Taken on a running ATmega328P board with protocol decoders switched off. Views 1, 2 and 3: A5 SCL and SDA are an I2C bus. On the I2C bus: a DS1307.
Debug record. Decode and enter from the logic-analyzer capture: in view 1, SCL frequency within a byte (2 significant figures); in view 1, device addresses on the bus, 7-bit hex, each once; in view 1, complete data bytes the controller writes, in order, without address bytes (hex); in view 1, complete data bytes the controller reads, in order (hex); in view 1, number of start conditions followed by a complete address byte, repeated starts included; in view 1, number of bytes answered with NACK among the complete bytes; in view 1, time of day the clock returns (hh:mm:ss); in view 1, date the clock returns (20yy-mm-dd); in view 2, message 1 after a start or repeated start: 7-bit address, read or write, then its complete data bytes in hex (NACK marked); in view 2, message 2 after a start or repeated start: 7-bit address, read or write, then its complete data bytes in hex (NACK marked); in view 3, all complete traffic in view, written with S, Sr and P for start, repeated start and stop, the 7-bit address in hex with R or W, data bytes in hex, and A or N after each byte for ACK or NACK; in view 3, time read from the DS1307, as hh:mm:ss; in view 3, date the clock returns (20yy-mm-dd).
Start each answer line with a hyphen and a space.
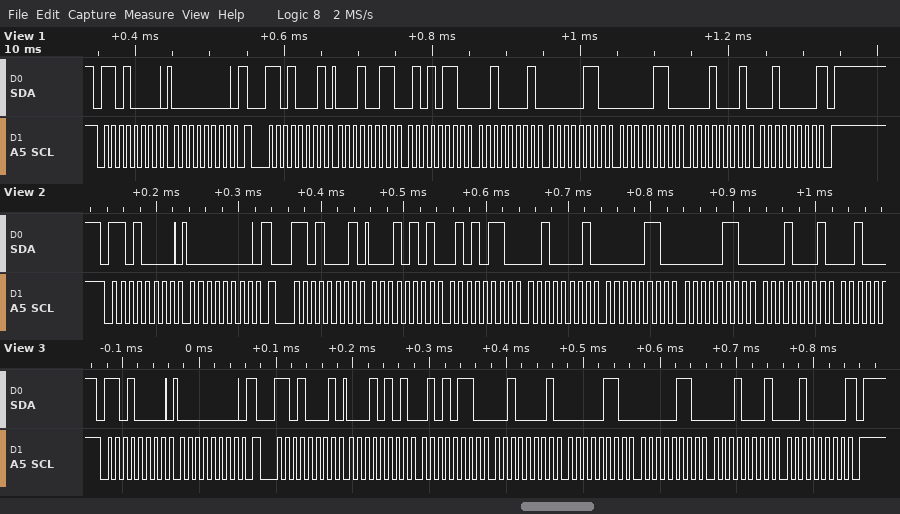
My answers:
- 100 kHz
- 0x68
- 00
- 13 56 21 06 06 11 20
- 2
- 1
- 21:56:13
- 2020-11-06
- 0x68 write: 00
- 0x68 read: 15 56 21 06 06 11
- S 68W A 00 A Sr 68R A 15 A 56 A 21 A 06 A 06 A 11 A 20 N P
- 21:56:15
- 2020-11-06
